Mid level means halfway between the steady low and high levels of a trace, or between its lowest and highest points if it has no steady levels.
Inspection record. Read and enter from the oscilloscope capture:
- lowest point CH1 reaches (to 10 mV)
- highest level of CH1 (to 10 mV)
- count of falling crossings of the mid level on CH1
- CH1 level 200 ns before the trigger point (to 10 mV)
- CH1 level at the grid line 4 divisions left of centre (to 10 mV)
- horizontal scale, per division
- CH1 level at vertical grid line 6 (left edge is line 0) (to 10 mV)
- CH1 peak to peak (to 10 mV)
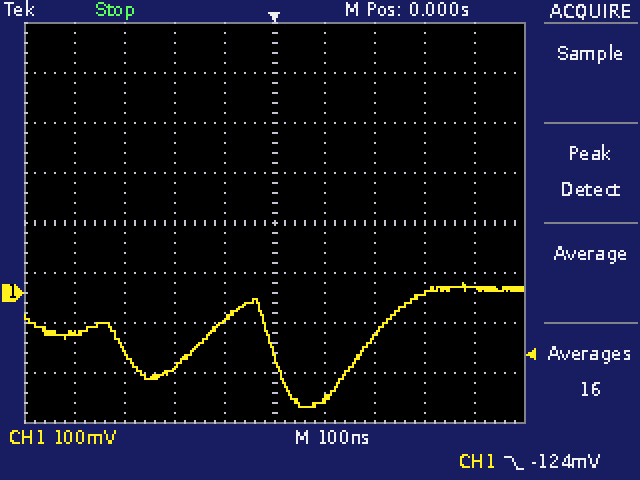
-230 mV
20 mV
2
-150 mV
-80 mV
100 ns
-210 mV
250 mV
